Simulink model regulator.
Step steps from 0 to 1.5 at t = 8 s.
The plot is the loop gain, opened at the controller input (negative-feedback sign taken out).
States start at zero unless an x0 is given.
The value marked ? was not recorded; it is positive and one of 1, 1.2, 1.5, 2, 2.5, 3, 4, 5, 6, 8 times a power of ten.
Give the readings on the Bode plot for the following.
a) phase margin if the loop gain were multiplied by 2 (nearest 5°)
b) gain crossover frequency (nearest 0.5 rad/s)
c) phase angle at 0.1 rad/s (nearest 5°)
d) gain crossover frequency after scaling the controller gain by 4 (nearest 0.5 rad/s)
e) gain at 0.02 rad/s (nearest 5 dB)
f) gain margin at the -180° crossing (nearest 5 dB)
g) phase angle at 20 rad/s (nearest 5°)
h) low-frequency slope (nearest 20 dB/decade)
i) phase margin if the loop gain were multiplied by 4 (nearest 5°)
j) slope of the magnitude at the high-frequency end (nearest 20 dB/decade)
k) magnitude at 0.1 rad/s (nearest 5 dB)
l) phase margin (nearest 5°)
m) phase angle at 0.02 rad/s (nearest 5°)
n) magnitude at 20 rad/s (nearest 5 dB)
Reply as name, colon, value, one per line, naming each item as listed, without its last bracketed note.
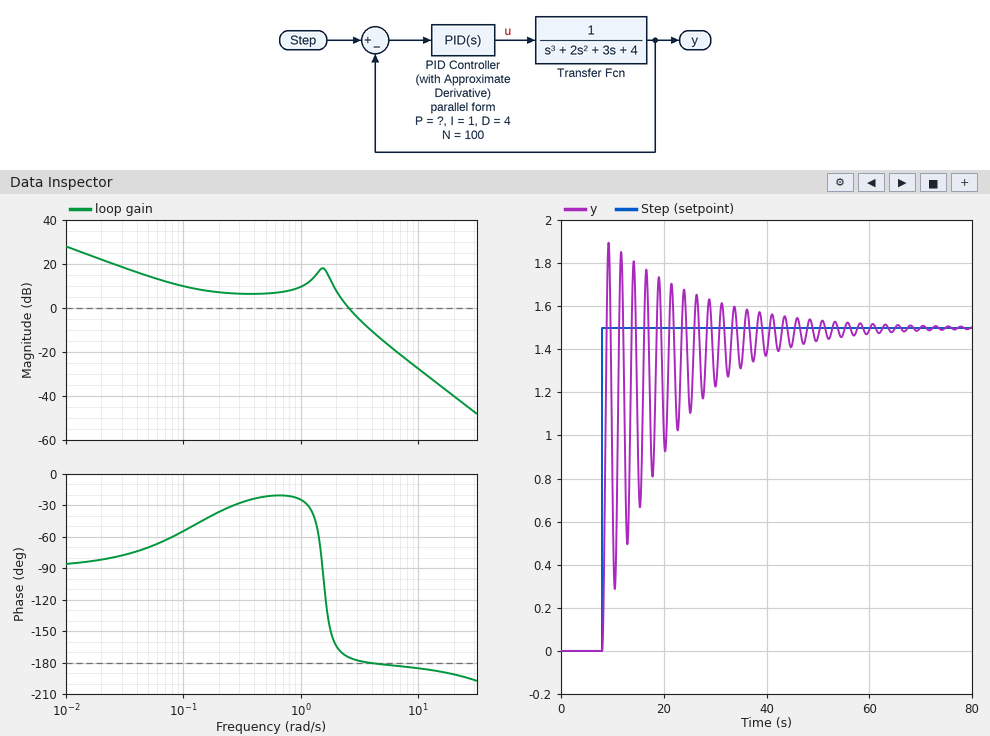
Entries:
phase margin if the loop gain were multiplied by 2: 0°
gain crossover frequency: 2.5 rad/s
phase angle at 0.1 rad/s: -55°
gain crossover frequency after scaling the controller gain by 4: 4.5 rad/s
gain at 0.02 rad/s: 20 dB
gain margin at the -180° crossing: 10 dB
phase angle at 20 rad/s: -190°
low-frequency slope: -20 dB/decade
phase margin if the loop gain were multiplied by 4: 0°
slope of the magnitude at the high-frequency end: -40 dB/decade
magnitude at 0.1 rad/s: 10 dB
phase margin: 5°
phase angle at 0.02 rad/s: -80°
magnitude at 20 rad/s: -40 dB
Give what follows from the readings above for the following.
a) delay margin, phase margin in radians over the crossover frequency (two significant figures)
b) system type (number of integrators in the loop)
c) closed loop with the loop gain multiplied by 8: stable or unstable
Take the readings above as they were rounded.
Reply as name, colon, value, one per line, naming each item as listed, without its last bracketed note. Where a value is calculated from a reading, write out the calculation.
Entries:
delay margin, phase margin in radians over the crossover frequency: 5 × π / 180 / 2.5 = 0.035 s
system type: 1
closed loop with the loop gain multiplied by 8: stable or unstable: unstable
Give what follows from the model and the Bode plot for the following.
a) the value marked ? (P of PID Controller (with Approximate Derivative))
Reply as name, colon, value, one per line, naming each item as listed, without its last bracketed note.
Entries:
the value marked ? (P of PID Controller (with Approximate Derivative)): 8
